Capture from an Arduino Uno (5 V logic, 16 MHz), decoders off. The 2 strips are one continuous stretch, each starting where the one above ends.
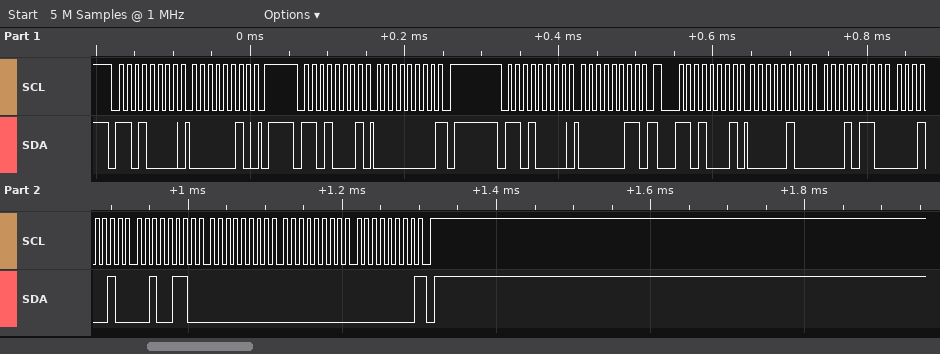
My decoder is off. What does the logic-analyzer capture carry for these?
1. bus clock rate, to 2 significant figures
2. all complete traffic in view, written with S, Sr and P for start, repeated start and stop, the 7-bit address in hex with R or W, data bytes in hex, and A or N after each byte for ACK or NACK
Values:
100 kHz
S 68W A 02 A P S 68R A 00 N P S 68W A 03 A Sr 68R A 04 A 16 A 12 A 26 A 00 A 00 A 00 N P
